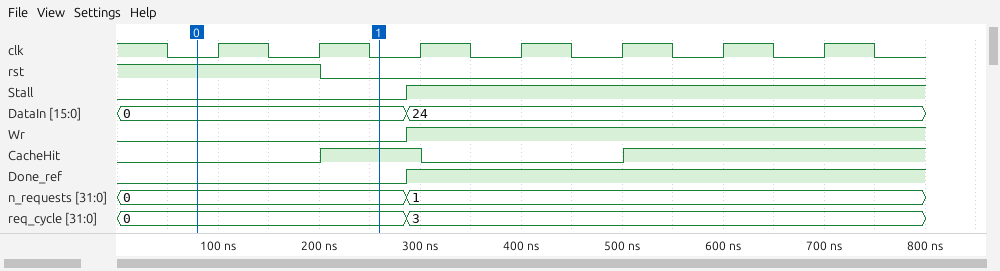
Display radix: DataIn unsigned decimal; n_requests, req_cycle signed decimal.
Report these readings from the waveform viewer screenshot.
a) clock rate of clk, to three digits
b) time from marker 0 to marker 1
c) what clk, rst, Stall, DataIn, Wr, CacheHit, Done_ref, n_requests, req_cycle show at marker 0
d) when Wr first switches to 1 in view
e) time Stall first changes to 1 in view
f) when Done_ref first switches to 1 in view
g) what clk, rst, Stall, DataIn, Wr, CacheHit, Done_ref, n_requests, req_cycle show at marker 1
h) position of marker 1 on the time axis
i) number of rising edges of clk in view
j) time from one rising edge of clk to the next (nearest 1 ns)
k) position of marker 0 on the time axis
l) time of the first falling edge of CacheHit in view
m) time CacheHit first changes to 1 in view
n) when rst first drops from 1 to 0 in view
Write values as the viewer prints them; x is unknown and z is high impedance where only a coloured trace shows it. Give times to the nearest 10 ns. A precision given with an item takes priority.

10.0 MHz
180 ns
clk=0, rst=1, Stall=0, DataIn=0, Wr=0, CacheHit=0, Done_ref=0, n_requests=0, req_cycle=0
290 ns
290 ns
290 ns
clk=0, rst=0, Stall=0, DataIn=0, Wr=0, CacheHit=1, Done_ref=0, n_requests=0, req_cycle=0
260 ns
7
100 ns
80 ns
300 ns
200 ns
200 ns
